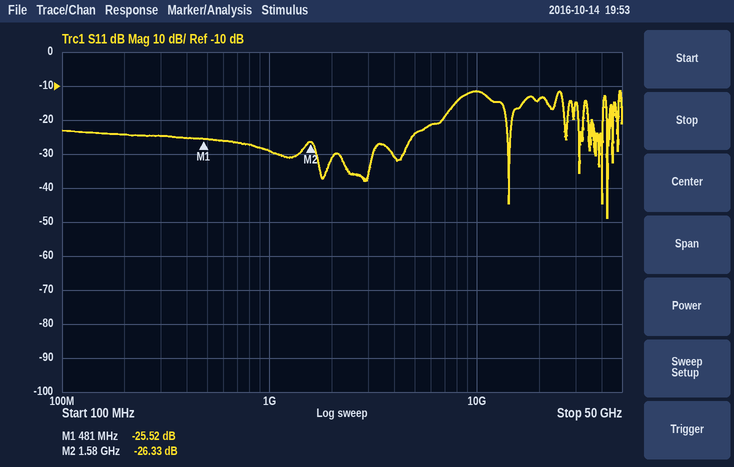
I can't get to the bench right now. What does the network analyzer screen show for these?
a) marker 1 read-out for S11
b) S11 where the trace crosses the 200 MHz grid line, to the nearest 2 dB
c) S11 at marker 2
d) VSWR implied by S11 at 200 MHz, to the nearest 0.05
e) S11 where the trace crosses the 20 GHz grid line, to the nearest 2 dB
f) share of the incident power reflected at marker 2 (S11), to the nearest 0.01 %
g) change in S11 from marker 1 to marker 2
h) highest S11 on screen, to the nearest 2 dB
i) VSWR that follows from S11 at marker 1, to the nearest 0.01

-25.52 dB
-24 dB
-26.33 dB
1.15
-14 dB
0.23 %
-0.81 dB
-12 dB
1.11
